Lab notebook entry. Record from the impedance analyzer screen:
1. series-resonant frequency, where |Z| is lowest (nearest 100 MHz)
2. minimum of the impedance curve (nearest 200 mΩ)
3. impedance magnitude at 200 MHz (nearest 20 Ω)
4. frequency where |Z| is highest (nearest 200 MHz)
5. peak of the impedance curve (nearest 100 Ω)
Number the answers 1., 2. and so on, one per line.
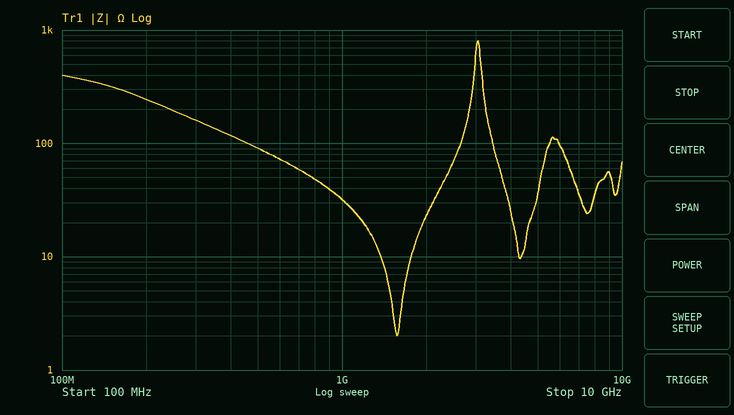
1. 1.6 GHz
2. 2.0 Ω
3. 240 Ω
4. 3.0 GHz
5. 800 Ω
